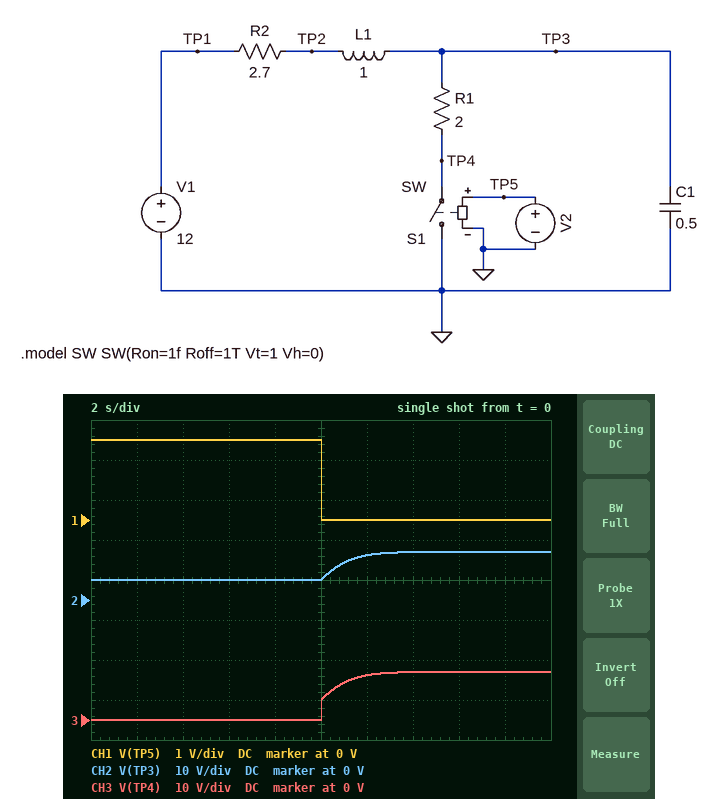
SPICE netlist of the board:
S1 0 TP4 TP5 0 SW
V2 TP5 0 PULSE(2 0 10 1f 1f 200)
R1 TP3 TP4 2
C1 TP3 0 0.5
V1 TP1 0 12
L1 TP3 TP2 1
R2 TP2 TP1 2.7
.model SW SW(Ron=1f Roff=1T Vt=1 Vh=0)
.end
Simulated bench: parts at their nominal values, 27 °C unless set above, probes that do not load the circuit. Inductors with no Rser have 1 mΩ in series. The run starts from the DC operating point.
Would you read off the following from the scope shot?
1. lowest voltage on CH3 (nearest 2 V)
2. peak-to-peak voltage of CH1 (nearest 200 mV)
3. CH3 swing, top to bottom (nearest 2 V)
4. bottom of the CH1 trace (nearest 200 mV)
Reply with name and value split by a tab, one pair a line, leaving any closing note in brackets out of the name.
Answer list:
lowest voltage on CH3	0 V
peak-to-peak voltage of CH1	2.0 V
CH3 swing, top to bottom	12 V
bottom of the CH1 trace	0 V
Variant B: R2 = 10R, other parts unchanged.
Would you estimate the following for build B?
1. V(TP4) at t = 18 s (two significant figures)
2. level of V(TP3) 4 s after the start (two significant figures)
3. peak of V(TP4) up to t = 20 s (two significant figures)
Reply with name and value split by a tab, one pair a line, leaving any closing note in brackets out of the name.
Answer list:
V(TP4) at t = 18 s	10 V
level of V(TP3) 4 s after the start	2.0 V
peak of V(TP4) up to t = 20 s	11 V
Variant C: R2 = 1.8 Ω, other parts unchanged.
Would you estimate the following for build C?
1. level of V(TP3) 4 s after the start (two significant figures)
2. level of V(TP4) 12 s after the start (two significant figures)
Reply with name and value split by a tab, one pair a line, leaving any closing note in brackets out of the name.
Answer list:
level of V(TP3) 4 s after the start	6.3 V
level of V(TP4) 12 s after the start	13 V
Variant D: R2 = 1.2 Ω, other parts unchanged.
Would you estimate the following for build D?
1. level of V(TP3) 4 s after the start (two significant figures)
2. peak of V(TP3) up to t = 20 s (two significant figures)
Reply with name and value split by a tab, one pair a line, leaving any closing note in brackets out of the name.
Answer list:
level of V(TP3) 4 s after the start	7.5 V
peak of V(TP3) up to t = 20 s	14 V
